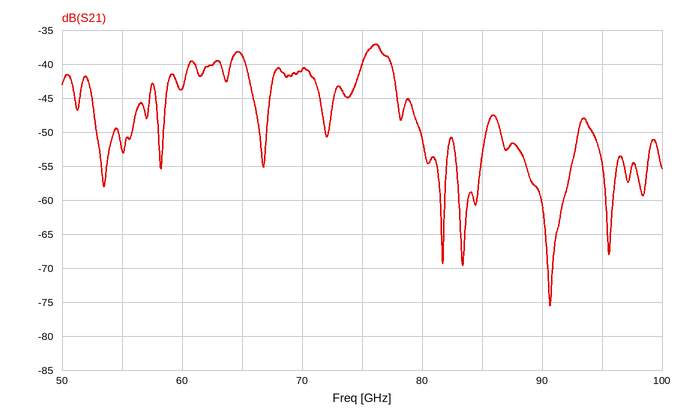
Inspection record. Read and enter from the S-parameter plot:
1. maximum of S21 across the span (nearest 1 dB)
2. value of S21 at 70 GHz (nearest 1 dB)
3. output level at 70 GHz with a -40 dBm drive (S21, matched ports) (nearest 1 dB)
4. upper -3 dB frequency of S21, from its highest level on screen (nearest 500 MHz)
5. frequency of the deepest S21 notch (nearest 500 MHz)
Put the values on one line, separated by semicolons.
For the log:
-37 dB; -41 dB; -81 dBm; 77.5 GHz; 90.5 GHz
